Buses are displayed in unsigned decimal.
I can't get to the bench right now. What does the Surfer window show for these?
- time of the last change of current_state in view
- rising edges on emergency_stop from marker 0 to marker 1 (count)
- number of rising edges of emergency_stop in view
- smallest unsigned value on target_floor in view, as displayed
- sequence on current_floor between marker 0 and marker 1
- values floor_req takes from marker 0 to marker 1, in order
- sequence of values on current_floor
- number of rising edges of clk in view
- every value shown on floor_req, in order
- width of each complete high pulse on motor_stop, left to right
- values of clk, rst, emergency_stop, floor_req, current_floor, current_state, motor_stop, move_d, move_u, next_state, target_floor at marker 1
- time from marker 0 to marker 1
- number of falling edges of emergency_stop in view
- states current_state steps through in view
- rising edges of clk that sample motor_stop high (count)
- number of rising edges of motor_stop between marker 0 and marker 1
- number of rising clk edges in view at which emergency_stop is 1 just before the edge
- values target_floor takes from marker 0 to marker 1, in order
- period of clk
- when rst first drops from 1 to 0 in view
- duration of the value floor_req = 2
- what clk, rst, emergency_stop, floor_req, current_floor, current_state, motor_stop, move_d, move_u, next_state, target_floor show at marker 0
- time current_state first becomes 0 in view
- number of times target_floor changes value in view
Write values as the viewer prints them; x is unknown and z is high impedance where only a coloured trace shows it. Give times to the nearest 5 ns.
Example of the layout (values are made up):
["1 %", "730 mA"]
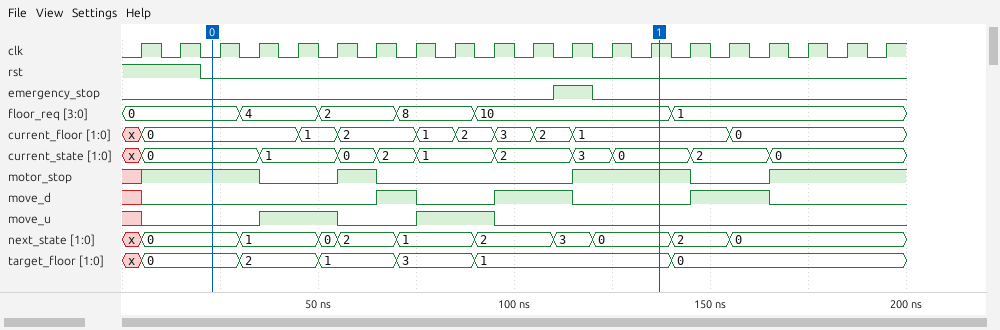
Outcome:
["165 ns", "1", "1", "0", "0, 1, 2, 1, 2, 3, 2, 1", "0, 4, 2, 8, 10", "x, 0, 1, 2, 1, 2, 3, 2, 1, 0", "20", "0, 4, 2, 8, 10, 1", "10 ns, 30 ns", "clk=1, rst=0, emergency_stop=0, floor_req=10, current_floor=1, current_state=0, motor_stop=1, move_d=0, move_u=0, next_state=0, target_floor=1", "115 ns", "1", "x, 0, 1, 0, 2, 1, 2, 3, 0, 2, 0", "10", "2", "1", "0, 2, 1, 3, 1", "10 ns", "20 ns", "20 ns", "clk=0, rst=0, emergency_stop=0, floor_req=0, current_floor=0, current_state=0, motor_stop=1, move_d=0, move_u=0, next_state=0, target_floor=0", "5 ns", "6"]
